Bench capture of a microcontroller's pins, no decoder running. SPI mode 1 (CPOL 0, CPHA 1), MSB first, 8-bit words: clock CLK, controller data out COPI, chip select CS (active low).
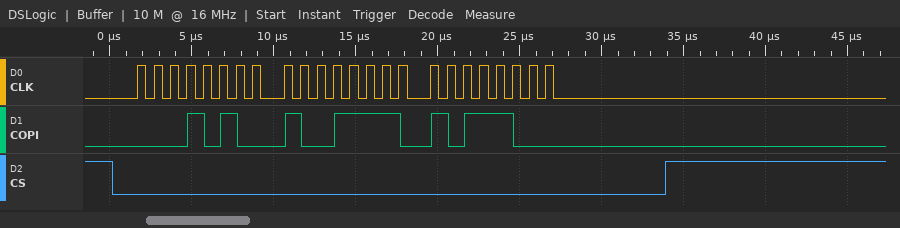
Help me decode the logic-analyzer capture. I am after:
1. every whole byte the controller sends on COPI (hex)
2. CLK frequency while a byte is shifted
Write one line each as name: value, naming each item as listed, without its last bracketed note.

every whole byte the controller sends on COPI: 14 9E B8
CLK frequency while a byte is shifted: 1 MHz
